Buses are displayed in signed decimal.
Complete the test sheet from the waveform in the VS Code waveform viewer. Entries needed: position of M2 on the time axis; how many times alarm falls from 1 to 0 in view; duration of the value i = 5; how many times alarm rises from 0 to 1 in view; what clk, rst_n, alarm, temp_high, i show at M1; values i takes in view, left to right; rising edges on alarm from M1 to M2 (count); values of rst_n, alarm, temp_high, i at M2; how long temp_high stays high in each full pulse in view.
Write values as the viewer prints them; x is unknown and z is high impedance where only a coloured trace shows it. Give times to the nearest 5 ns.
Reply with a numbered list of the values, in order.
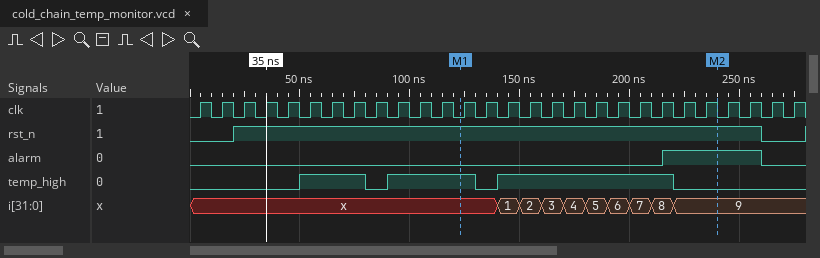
1. 240 ns
2. 1
3. 10 ns
4. 1
5. clk=0, rst_n=1, alarm=0, temp_high=1, i=x
6. x, 1, 2, 3, 4, 5, 6, 7, 8, 9
7. 1
8. rst_n=1, alarm=1, temp_high=0, i=9
9. 30 ns, 40 ns, 80 ns
